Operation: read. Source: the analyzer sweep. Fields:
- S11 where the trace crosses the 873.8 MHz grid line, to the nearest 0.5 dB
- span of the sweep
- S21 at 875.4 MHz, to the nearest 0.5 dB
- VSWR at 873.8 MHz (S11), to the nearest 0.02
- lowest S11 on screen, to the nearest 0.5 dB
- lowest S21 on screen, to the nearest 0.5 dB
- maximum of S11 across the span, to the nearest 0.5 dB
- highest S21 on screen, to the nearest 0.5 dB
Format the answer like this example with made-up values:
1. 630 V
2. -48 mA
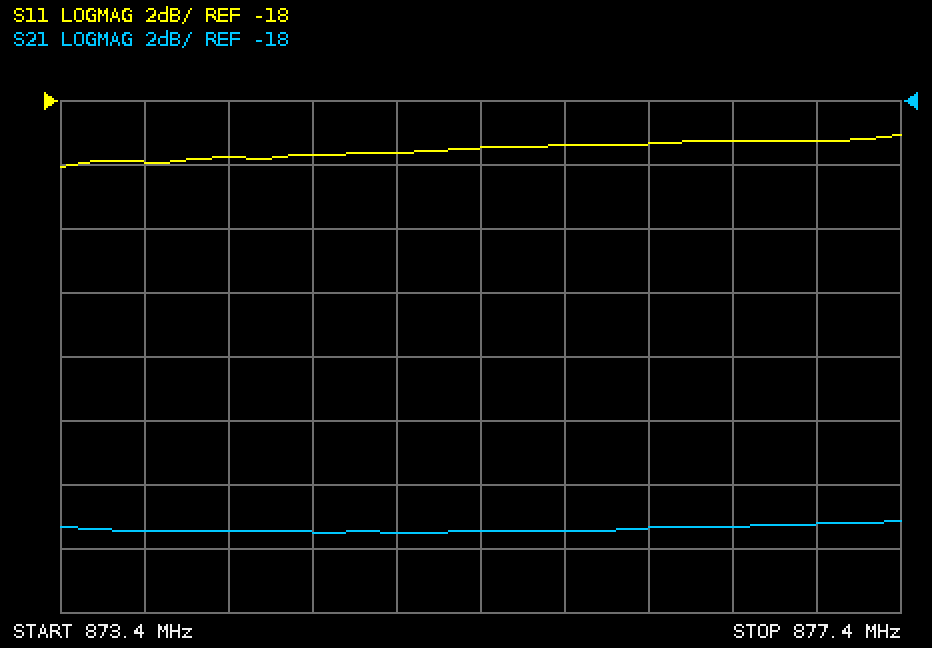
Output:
1. -20.0 dB
2. 4 MHz
3. -31.5 dB
4. 1.22
5. -20.0 dB
6. -31.5 dB
7. -19.0 dB
8. -31.0 dB
